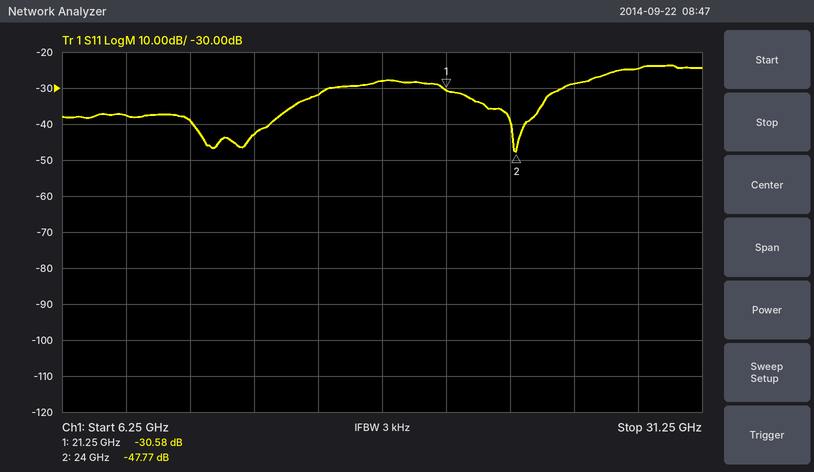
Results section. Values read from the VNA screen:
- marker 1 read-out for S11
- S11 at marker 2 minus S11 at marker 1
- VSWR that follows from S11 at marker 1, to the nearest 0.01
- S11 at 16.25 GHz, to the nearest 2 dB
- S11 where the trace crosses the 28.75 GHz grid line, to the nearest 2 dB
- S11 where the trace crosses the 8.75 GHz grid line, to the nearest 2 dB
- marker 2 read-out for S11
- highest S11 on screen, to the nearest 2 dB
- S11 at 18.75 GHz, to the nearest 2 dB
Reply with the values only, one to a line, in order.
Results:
-30.58 dB
-17.19 dB
1.06
-32 dB
-24 dB
-38 dB
-47.77 dB
-24 dB
-28 dB
